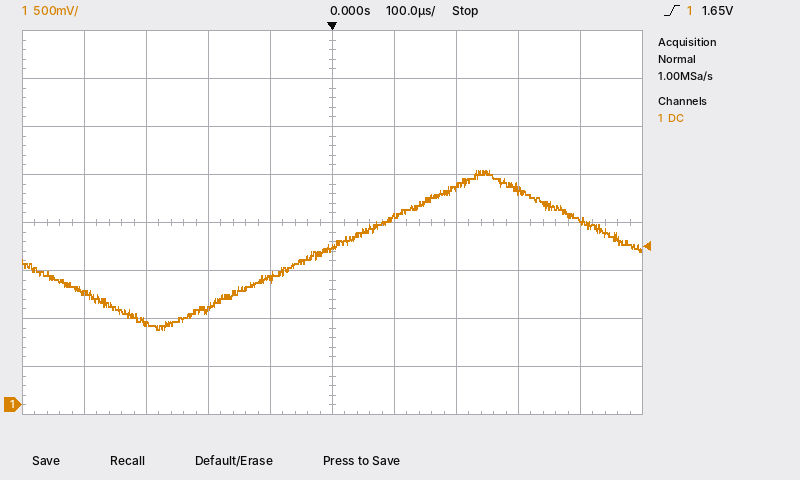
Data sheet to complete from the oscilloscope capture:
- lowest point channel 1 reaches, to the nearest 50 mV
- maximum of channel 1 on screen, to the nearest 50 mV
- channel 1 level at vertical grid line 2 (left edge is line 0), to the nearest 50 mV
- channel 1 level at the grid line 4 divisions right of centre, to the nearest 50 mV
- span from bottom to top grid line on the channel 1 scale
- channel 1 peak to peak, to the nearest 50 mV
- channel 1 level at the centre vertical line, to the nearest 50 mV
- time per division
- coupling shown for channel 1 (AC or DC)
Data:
800 mV
2.45 V
850 mV
1.90 V
4 V
1.65 V
1.65 V
100 µs
DC
